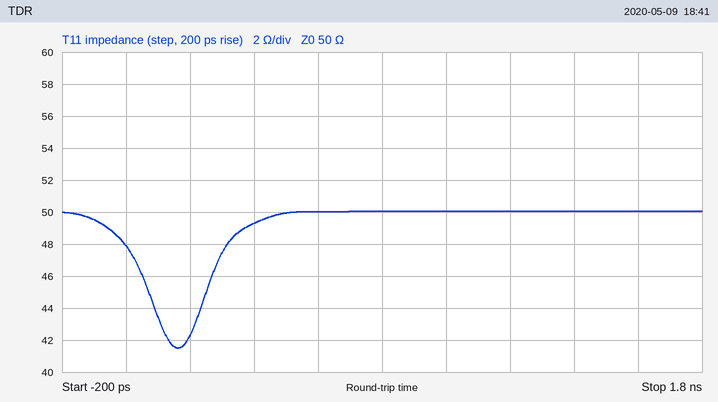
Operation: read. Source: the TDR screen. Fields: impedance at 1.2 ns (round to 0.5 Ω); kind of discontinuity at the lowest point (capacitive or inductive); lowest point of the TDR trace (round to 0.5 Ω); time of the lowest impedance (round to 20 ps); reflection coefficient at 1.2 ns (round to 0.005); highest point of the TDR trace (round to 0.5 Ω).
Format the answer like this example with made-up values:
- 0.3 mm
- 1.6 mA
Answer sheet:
- 50.0 Ω
- capacitive
- 41.5 Ω
- 160 ps
- 0.000
- 50.0 Ω
